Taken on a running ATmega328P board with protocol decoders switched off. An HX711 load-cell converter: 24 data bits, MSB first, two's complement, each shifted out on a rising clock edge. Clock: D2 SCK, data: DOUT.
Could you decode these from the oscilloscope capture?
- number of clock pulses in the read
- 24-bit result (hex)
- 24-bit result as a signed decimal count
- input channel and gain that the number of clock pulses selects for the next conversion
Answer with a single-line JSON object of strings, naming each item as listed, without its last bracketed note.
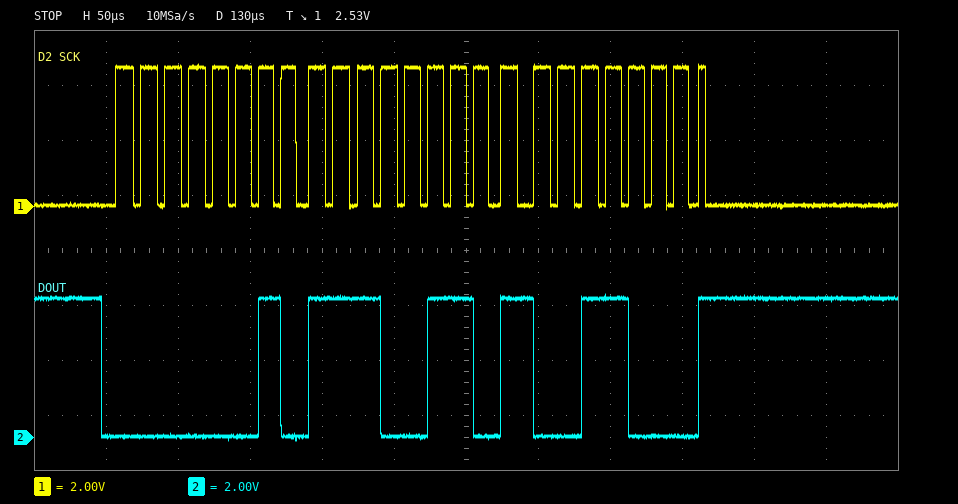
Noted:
{"number of clock pulses in the read": "25", "24-bit result": "0x02E698", "24-bit result as a signed decimal count": "190104", "input channel and gain that the number of clock pulses selects for the next conversion": "channel A, gain 128"}
